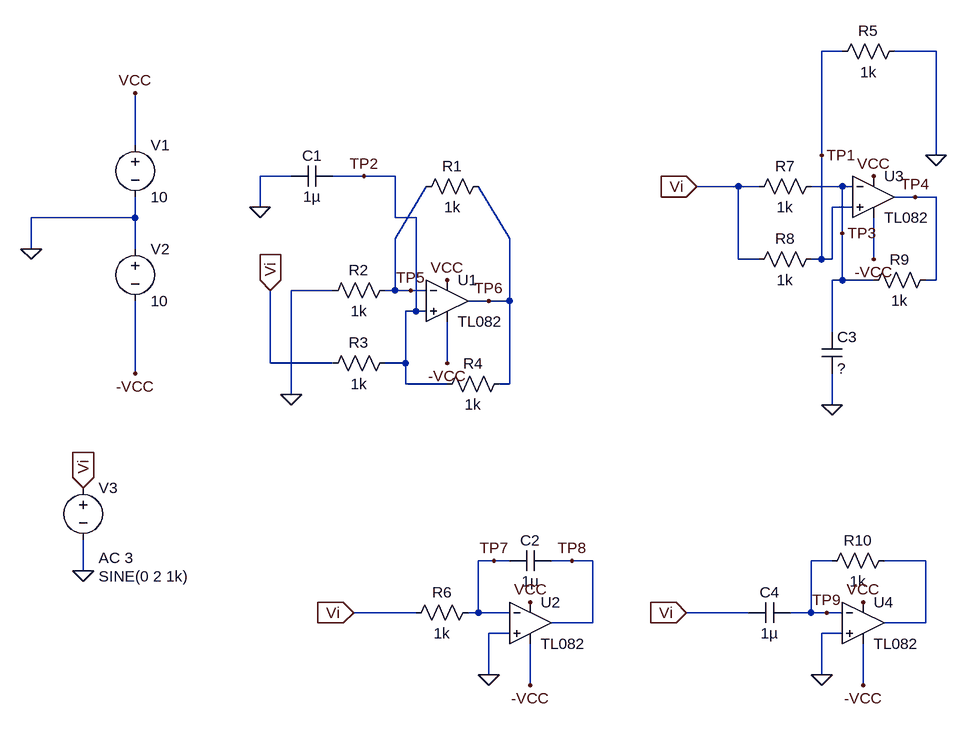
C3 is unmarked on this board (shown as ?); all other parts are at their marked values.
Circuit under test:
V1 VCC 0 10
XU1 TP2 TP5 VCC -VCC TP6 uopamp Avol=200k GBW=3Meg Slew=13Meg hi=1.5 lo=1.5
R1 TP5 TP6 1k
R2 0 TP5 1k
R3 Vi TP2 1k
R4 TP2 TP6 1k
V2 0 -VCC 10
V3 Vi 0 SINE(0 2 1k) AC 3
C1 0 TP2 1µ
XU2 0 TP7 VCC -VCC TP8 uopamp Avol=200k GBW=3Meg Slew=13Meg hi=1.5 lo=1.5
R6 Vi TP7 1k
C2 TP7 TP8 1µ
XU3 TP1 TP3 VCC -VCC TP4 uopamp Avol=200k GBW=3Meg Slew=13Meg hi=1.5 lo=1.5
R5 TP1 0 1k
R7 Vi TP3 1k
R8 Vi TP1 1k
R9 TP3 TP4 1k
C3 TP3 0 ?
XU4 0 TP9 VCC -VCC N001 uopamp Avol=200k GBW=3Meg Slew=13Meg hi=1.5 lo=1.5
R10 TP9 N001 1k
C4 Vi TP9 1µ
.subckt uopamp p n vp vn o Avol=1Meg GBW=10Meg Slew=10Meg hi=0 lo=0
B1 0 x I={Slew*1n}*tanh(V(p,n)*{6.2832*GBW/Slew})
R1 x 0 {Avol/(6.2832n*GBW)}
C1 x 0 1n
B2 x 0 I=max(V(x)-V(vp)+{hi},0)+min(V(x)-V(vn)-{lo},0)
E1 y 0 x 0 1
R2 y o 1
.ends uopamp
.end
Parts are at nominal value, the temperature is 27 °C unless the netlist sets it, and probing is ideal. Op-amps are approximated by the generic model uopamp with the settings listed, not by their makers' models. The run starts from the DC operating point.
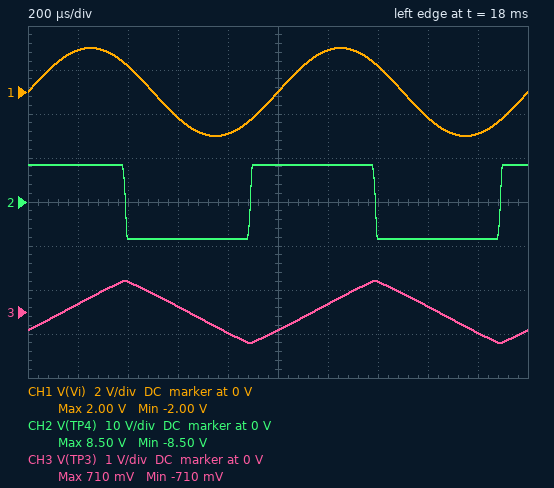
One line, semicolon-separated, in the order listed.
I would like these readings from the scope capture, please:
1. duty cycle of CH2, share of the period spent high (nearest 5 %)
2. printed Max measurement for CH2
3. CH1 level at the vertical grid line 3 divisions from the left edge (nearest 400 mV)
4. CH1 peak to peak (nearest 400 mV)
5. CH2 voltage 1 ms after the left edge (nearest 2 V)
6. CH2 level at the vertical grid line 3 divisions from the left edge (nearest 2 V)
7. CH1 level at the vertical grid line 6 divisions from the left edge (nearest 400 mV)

50 %; 8.50 V; -1.2 V; 4.0 V; 8 V; -8 V; 2.0 V
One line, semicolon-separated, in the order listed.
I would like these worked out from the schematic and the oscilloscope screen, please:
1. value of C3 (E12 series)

3.3 µF
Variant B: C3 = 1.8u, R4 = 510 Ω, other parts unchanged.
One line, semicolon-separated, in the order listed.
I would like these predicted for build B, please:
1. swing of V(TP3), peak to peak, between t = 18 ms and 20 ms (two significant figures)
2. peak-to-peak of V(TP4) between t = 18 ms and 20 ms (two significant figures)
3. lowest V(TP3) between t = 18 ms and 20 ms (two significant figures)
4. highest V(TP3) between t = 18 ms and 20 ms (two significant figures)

2.1 V; 17 V; -1.0 V; 1.0 V
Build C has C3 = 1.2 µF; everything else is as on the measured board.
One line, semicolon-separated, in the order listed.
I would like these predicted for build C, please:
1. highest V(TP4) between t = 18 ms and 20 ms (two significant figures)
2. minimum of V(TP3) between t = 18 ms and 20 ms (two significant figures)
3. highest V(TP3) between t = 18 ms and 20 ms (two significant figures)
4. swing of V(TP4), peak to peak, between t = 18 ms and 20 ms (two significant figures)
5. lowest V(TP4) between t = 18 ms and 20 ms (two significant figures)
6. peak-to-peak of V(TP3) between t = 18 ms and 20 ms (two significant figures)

7.6 V; -1.0 V; 1.0 V; 15 V; -7.6 V; 2.0 V
